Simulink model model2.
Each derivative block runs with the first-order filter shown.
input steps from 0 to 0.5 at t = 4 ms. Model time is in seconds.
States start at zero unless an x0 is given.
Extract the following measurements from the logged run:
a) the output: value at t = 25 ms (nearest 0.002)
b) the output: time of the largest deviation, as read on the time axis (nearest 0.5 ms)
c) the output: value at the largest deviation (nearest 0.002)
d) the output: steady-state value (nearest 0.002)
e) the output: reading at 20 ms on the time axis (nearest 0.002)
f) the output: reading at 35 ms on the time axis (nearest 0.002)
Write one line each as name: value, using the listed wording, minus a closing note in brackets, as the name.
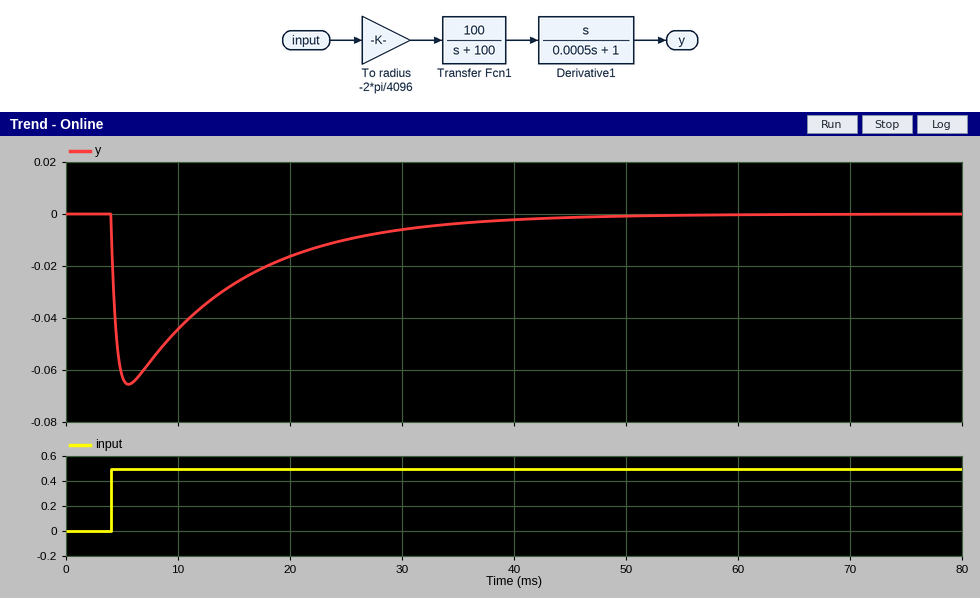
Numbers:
the output: value at t = 25 ms: -0.010
the output: time of the largest deviation, as read on the time axis: 5.5 ms
the output: value at the largest deviation: -0.066
the output: steady-state value: 0.000
the output: reading at 20 ms on the time axis: -0.016
the output: reading at 35 ms on the time axis: -0.004
